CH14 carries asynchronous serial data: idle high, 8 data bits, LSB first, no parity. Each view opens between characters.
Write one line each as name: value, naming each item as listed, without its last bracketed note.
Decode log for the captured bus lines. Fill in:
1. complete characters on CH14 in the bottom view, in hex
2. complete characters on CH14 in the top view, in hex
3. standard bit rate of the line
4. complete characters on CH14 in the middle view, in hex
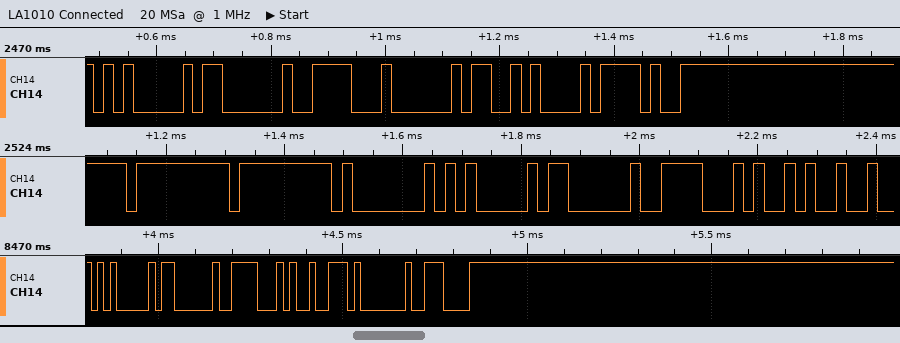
complete characters on CH14 in the bottom view, in hex: 05, 03, 1E, C9, 01, 0E
complete characters on CH14 in the top view, in hex: 05, 03, 1E, A0, 0A, 2F
standard bit rate of the line: 57600 baud
complete characters on CH14 in the middle view, in hex: FF, FF, 01, 05, 03, 1E, 29
